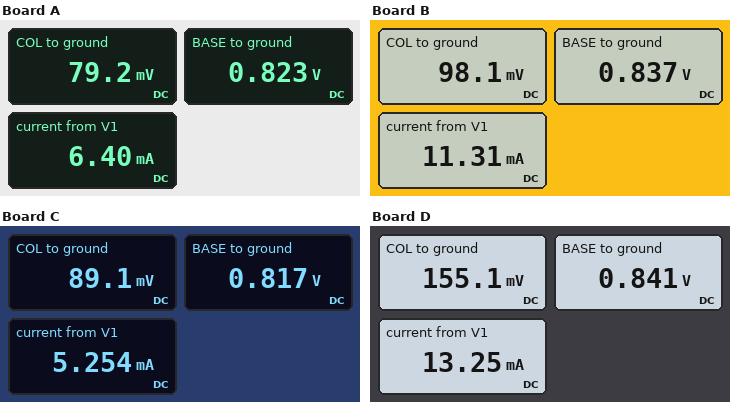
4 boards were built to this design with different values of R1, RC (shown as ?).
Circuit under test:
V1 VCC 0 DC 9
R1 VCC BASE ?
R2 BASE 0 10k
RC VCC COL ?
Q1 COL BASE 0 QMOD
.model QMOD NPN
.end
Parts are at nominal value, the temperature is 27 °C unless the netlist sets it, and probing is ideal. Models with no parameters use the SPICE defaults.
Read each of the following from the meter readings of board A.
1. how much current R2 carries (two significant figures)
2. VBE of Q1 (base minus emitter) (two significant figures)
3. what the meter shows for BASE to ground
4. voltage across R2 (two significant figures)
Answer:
82 µA
820 mV
0.823 V
820 mV
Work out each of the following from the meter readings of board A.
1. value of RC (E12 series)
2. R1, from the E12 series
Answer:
1.5 kΩ
18 kΩ
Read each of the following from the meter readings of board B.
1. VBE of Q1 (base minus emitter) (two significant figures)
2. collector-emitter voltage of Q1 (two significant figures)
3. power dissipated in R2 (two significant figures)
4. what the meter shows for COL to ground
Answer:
840 mV
98 mV
70 µW
98.1 mV
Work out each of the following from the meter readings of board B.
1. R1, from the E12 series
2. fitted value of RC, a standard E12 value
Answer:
18 kΩ
820 Ω
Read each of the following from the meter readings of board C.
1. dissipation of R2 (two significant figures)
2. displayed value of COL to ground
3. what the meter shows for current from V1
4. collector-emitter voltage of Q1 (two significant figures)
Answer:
67 µW
89.1 mV
5.254 mA
89 mV
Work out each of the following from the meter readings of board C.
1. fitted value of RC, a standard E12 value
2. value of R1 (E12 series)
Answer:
1.8 kΩ
27 kΩ
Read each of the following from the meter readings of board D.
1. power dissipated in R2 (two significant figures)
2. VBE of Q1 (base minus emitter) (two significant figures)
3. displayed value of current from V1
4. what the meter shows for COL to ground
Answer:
71 µW
840 mV
13.25 mA
155.1 mV
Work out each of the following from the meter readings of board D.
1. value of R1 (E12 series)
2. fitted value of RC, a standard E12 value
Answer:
33 kΩ
680 Ω
